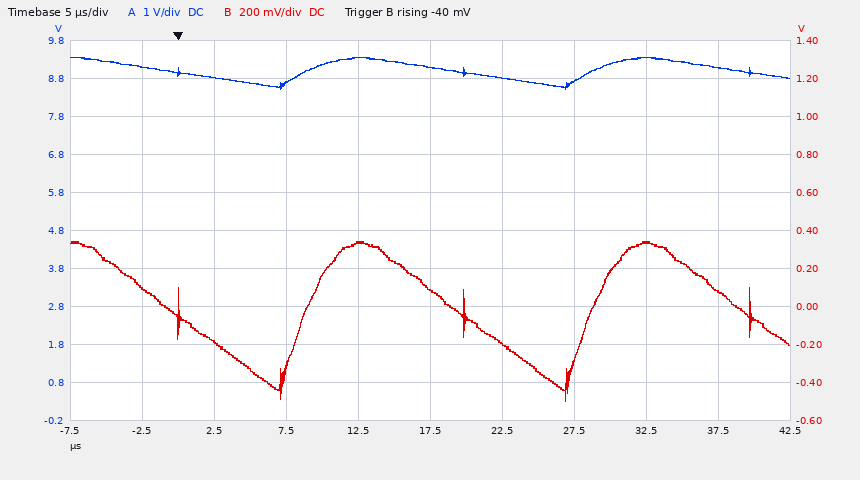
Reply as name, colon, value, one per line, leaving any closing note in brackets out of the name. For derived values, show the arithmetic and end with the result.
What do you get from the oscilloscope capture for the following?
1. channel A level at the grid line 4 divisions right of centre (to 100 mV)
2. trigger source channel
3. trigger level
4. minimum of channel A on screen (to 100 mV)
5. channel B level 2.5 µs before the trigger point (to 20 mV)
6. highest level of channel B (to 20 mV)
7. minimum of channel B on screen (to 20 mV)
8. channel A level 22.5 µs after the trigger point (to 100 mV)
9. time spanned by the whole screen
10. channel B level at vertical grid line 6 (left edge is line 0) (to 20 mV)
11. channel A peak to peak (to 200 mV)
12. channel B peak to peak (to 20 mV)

channel A level at the grid line 4 divisions right of centre: 9.1 V
trigger source channel: channel B
trigger level: -40 mV
minimum of channel A on screen: 8.5 V
channel B level 2.5 µs before the trigger point: 100 mV
highest level of channel B: 340 mV
minimum of channel B on screen: -500 mV
channel A level 22.5 µs after the trigger point: 8.8 V
time spanned by the whole screen: 50 µs
channel B level at vertical grid line 6 (left edge is line 0): -200 mV
channel A peak to peak: 800 mV
channel B peak to peak: 340 mV − (-500 mV) = 840 mV
